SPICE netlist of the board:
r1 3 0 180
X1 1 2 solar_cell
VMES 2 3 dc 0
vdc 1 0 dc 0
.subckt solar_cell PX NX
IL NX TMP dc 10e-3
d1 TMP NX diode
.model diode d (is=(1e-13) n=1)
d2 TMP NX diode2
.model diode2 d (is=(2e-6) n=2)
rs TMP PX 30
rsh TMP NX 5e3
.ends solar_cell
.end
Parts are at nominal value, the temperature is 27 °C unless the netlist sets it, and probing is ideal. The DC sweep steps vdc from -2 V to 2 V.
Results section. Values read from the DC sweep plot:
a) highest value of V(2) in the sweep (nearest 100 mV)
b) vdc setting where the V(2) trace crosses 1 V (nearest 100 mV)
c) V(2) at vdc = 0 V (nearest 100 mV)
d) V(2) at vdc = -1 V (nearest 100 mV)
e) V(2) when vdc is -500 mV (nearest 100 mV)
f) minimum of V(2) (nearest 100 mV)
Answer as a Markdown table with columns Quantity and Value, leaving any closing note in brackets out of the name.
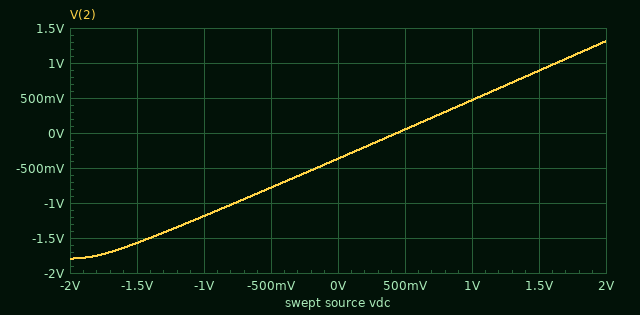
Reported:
| Quantity | Value |
|---|---|
| highest value of V(2) in the sweep | 1.3 V |
| vdc setting where the V(2) trace crosses 1 V | 1.6 V |
| V(2) at vdc = 0 V | -400 mV |
| V(2) at vdc = -1 V | -1.2 V |
| V(2) when vdc is -500 mV | -800 mV |
| minimum of V(2) | -1.8 V |
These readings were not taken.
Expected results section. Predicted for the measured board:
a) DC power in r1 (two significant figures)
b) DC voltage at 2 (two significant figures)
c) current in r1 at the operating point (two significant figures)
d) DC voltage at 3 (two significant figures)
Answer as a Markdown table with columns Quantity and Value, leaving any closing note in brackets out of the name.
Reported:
| Quantity | Value |
|---|---|
| DC power in r1 | 750 µW |
| DC voltage at 2 | -370 mV |
| current in r1 at the operating point | 2.0 mA |
| DC voltage at 3 | -370 mV |
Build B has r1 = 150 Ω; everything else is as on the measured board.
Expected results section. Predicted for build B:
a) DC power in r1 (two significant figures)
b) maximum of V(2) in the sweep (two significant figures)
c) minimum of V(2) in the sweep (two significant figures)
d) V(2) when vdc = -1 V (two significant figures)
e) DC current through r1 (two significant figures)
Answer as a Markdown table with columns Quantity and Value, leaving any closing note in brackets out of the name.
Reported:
| Quantity | Value |
|---|---|
| DC power in r1 | 840 µW |
| maximum of V(2) in the sweep | 1.3 V |
| minimum of V(2) in the sweep | -1.5 V |
| V(2) when vdc = -1 V | -1.1 V |
| DC current through r1 | 2.4 mA |
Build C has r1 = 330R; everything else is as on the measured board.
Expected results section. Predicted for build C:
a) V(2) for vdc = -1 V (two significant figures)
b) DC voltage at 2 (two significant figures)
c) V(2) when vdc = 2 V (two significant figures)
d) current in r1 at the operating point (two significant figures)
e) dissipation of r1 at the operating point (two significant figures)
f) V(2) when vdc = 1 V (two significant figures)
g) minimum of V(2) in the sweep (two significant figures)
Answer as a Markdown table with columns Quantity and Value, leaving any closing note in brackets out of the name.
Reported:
| Quantity | Value |
|---|---|
| V(2) for vdc = -1 V | -1.3 V |
| DC voltage at 2 | -400 mV |
| V(2) when vdc = 2 V | 1.4 V |
| current in r1 at the operating point | 1.2 mA |
| dissipation of r1 at the operating point | 480 µW |
| V(2) when vdc = 1 V | 510 mV |
| minimum of V(2) in the sweep | -2.2 V |
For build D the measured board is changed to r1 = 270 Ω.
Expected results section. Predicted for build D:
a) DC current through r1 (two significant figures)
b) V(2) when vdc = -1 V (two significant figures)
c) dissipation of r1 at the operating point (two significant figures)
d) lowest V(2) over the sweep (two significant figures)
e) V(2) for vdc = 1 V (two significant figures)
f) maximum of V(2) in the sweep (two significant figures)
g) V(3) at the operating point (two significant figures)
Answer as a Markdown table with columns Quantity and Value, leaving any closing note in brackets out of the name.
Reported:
| Quantity | Value |
|---|---|
| DC current through r1 | 1.4 mA |
| V(2) when vdc = -1 V | -1.3 V |
| dissipation of r1 at the operating point | 560 µW |
| lowest V(2) over the sweep | -2.1 V |
| V(2) for vdc = 1 V | 500 mV |
| maximum of V(2) in the sweep | 1.4 V |
| V(3) at the operating point | -390 mV |
